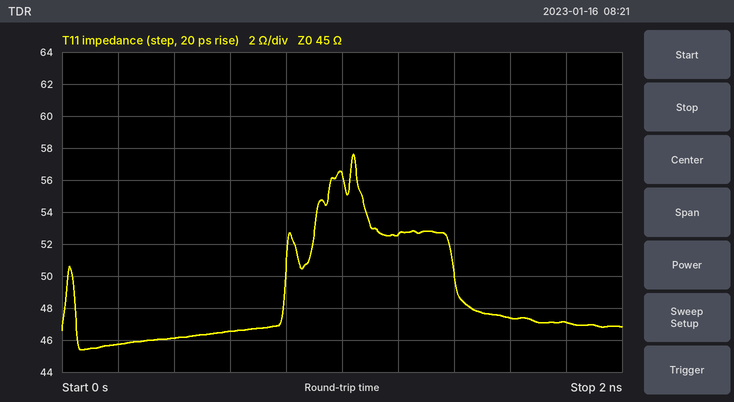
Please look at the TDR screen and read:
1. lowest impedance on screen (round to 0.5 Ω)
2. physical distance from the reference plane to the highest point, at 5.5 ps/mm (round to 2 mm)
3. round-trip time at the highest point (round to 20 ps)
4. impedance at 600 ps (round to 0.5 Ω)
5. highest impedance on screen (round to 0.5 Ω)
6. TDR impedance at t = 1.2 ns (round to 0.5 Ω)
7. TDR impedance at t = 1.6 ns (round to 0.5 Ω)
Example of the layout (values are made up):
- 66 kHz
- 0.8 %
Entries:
- 45.5 Ω
- 94 mm
- 1.04 ns
- 46.5 Ω
- 57.5 Ω
- 52.5 Ω
- 47.5 Ω
